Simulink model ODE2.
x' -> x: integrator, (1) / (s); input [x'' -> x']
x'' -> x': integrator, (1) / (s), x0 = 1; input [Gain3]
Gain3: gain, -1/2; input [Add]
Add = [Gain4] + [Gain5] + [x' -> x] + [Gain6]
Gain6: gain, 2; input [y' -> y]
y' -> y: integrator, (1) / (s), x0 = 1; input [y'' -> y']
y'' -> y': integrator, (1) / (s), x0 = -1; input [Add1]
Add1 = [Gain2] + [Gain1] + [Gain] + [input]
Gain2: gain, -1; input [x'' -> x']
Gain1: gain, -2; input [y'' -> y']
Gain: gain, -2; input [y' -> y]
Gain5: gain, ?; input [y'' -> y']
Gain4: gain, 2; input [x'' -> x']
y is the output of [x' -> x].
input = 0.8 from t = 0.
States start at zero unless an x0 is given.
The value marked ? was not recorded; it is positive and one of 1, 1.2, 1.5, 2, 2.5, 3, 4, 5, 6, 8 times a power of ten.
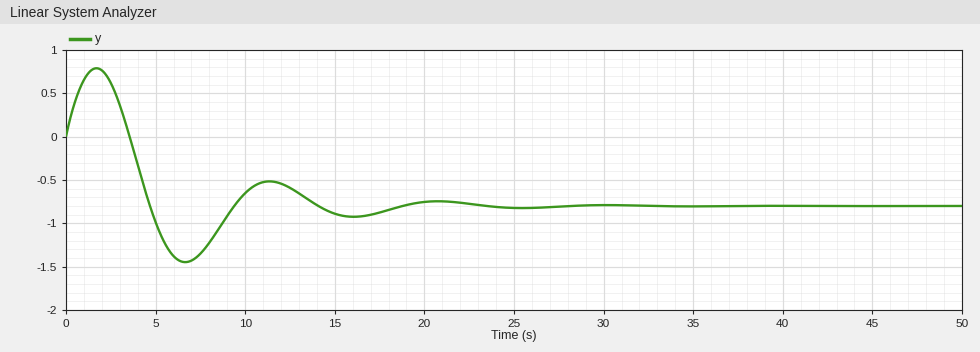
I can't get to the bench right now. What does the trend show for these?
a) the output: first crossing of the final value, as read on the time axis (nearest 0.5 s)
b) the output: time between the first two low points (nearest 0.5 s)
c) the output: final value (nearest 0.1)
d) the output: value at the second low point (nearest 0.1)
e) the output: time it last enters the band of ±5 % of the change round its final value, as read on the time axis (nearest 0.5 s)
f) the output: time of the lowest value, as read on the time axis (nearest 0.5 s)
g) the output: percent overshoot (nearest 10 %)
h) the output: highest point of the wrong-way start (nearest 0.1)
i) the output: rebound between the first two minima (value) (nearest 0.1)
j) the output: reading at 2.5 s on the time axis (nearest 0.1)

4.5 s
9.5 s
-0.8
-0.9
22.0 s
6.5 s
80 %
0.8
-0.5
0.6
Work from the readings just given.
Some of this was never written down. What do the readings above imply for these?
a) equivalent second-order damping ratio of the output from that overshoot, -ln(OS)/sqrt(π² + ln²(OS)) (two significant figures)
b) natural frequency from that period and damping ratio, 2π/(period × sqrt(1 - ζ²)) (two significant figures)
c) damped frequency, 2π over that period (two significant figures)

0.071
0.66 rad/s
0.66 rad/s
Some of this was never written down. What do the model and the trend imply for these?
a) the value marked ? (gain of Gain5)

2
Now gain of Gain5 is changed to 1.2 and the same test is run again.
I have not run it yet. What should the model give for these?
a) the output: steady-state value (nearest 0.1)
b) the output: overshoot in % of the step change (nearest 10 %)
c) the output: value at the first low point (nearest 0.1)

-0.8
60 %
-1.3
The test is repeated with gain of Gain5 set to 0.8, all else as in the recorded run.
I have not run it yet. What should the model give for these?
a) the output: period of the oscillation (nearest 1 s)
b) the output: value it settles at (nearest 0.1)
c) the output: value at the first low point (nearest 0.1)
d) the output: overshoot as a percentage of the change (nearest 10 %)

11 s
-0.8
-1.2
50 %
